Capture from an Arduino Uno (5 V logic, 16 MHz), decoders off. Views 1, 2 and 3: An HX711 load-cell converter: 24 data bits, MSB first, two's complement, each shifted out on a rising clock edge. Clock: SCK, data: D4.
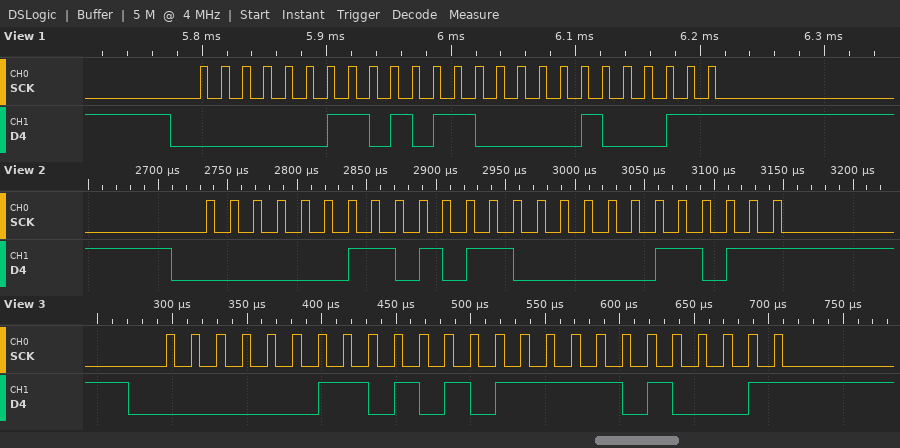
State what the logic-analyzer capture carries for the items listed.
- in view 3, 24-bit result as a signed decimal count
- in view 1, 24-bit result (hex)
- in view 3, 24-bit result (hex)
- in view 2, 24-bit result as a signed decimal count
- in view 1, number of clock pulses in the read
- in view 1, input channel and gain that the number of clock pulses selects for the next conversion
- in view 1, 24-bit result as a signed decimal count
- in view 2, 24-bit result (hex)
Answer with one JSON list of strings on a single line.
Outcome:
["219089", "0x035823", "0x0357D1", "219163", "25", "channel A, gain 128", "219171", "0x03581B"]
